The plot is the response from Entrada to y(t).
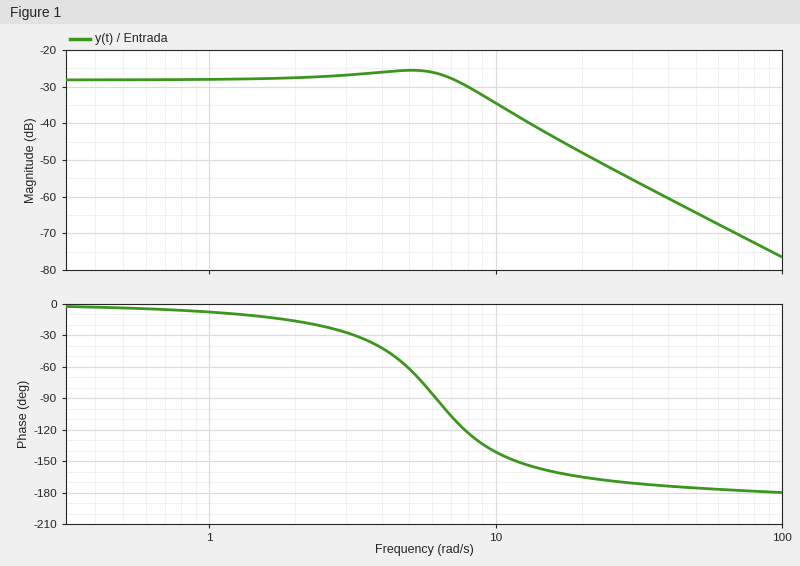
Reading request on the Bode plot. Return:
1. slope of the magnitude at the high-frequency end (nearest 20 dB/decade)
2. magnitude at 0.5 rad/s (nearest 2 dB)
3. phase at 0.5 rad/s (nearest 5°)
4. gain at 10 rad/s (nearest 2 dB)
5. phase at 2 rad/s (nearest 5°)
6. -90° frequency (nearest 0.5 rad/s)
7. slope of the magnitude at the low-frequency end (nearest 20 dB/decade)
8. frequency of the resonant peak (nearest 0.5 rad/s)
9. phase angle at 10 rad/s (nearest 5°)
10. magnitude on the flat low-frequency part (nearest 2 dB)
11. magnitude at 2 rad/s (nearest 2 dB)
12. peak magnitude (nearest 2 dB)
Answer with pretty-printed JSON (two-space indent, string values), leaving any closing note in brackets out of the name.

{
  "slope of the magnitude at the high-frequency end": "-40 dB/decade",
  "magnitude at 0.5 rad/s": "-28 dB",
  "phase at 0.5 rad/s": "-5°",
  "gain at 10 rad/s": "-34 dB",
  "phase at 2 rad/s": "-15°",
  "-90° frequency": "6.0 rad/s",
  "slope of the magnitude at the low-frequency end": "0 dB/decade",
  "frequency of the resonant peak": "5.0 rad/s",
  "phase angle at 10 rad/s": "-140°",
  "magnitude on the flat low-frequency part": "-28 dB",
  "magnitude at 2 rad/s": "-28 dB",
  "peak magnitude": "-26 dB"
}
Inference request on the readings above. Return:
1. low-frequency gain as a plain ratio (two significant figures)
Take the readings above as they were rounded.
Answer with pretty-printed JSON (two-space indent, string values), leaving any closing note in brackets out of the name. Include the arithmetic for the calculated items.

{
  "low-frequency gain as a plain ratio": "10^(-28 / 20) = 0.040"
}
